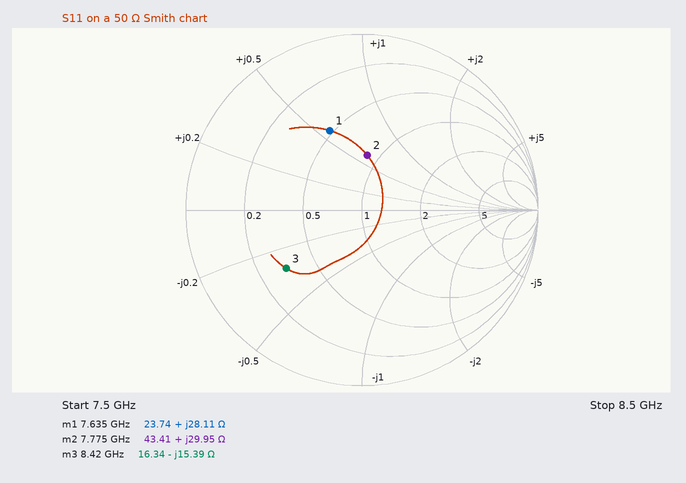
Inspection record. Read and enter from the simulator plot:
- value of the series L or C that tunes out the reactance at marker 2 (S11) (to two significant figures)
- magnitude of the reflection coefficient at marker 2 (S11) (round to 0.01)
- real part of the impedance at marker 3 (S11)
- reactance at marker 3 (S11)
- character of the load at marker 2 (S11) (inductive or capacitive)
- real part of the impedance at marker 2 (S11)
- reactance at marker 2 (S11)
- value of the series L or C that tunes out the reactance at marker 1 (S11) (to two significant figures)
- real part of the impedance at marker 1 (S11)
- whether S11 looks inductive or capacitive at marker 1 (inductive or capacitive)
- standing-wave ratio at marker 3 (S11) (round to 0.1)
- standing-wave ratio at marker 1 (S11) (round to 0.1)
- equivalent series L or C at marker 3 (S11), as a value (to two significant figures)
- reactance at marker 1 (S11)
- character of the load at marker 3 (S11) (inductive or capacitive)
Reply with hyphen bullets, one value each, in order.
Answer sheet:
- 680 fF
- 0.31
- 16.34 Ω
- -15.39 Ω
- inductive
- 43.41 Ω
- +29.95 Ω
- 740 fF
- 23.74 Ω
- inductive
- 3.4
- 2.9
- 1.2 pF
- +28.11 Ω
- capacitive
